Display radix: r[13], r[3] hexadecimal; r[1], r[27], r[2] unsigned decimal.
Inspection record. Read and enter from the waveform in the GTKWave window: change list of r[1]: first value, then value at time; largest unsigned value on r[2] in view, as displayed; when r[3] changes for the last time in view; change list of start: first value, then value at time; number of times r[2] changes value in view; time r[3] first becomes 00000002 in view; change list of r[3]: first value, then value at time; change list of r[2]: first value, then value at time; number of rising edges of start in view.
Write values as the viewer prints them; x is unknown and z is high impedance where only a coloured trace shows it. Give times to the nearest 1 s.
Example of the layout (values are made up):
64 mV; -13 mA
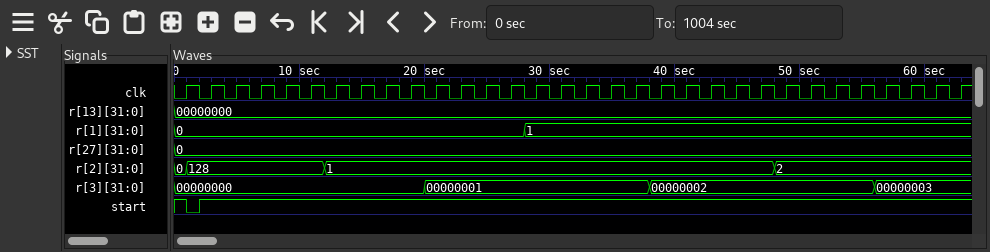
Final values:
0, 1 at 28 s; 128; 56 s; 1, 0 at 1 s, 1 at 2 s; 3; 38 s; 00000000, 00000001 at 20 s, 00000002 at 38 s, 00000003 at 56 s; 0, 128 at 1 s, 1 at 12 s, 2 at 48 s; 1
